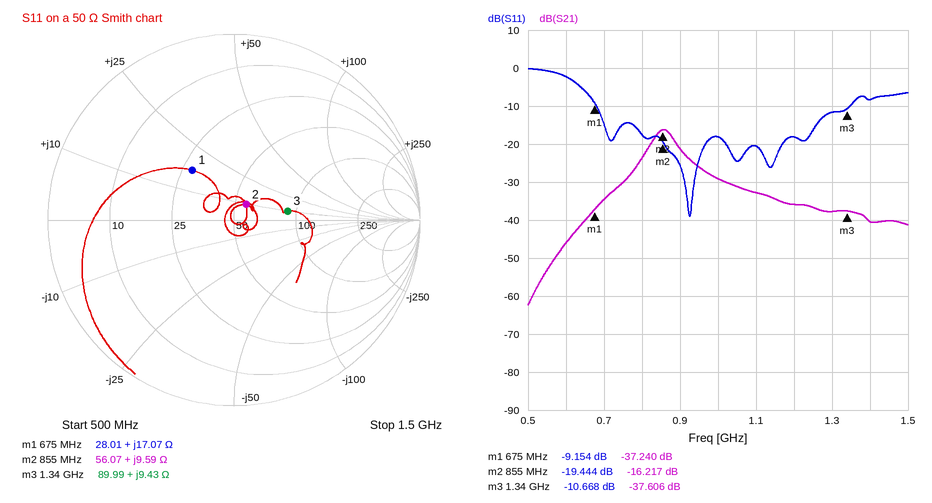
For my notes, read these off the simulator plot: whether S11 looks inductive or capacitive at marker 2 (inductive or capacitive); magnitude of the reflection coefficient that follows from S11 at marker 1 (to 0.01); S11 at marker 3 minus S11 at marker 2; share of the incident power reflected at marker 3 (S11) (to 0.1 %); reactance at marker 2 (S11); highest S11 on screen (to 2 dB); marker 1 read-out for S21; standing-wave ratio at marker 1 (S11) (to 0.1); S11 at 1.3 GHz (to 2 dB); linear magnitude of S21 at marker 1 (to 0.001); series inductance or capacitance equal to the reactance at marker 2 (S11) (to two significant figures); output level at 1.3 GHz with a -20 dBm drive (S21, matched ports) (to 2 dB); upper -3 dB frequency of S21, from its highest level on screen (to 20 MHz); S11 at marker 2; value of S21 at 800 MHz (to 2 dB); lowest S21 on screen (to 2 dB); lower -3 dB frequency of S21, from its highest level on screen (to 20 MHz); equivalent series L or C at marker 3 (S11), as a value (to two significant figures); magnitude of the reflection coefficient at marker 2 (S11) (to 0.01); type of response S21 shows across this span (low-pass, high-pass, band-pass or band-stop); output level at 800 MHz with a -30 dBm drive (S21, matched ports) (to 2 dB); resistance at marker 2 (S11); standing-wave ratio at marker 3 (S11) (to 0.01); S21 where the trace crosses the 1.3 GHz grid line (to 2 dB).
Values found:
inductive
0.35
8.776 dB
8.6 %
+9.59 Ω
0 dB
-37.240 dB
2.1
-12 dB
0.014
1.8 nH
-58 dBm
880 MHz
-19.444 dB
-24 dB
-62 dB
820 MHz
1.1 nH
0.11
band-pass
-54 dBm
56.07 Ω
1.83
-38 dB
